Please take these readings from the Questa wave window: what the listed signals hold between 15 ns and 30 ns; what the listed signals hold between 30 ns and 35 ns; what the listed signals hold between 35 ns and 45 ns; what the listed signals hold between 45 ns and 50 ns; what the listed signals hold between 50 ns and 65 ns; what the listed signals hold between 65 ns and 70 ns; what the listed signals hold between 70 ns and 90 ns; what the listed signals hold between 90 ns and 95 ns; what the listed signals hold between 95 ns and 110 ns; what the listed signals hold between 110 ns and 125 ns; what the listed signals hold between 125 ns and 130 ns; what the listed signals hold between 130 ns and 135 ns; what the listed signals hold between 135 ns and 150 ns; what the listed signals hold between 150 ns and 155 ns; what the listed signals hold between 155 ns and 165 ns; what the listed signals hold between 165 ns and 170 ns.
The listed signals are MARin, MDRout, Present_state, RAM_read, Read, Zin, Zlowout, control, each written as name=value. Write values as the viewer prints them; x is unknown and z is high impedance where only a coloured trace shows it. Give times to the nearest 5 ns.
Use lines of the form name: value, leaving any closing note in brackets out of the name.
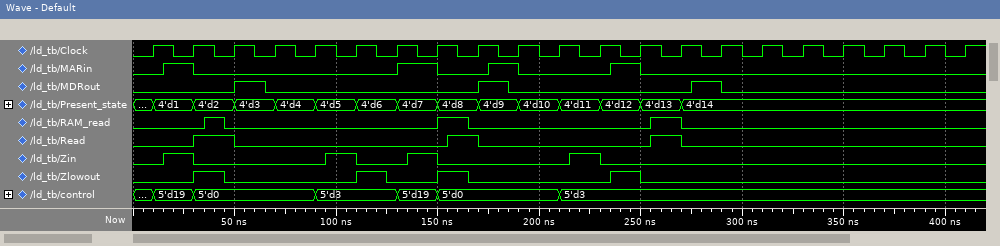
what the listed signals hold between 15 ns and 30 ns: MARin=1, MDRout=0, Present_state=4'd1, RAM_read=0, Read=0, Zin=1, Zlowout=0, control=5'd19
what the listed signals hold between 30 ns and 35 ns: MARin=0, MDRout=0, Present_state=4'd2, RAM_read=0, Read=1, Zin=0, Zlowout=1, control=5'd0
what the listed signals hold between 35 ns and 45 ns: MARin=0, MDRout=0, Present_state=4'd2, RAM_read=1, Read=1, Zin=0, Zlowout=1, control=5'd0
what the listed signals hold between 45 ns and 50 ns: MARin=0, MDRout=0, Present_state=4'd2, RAM_read=0, Read=1, Zin=0, Zlowout=0, control=5'd0
what the listed signals hold between 50 ns and 65 ns: MARin=0, MDRout=1, Present_state=4'd3, RAM_read=0, Read=0, Zin=0, Zlowout=0, control=5'd0
what the listed signals hold between 65 ns and 70 ns: MARin=0, MDRout=0, Present_state=4'd3, RAM_read=0, Read=0, Zin=0, Zlowout=0, control=5'd0
what the listed signals hold between 70 ns and 90 ns: MARin=0, MDRout=0, Present_state=4'd4, RAM_read=0, Read=0, Zin=0, Zlowout=0, control=5'd0
what the listed signals hold between 90 ns and 95 ns: MARin=0, MDRout=0, Present_state=4'd5, RAM_read=0, Read=0, Zin=0, Zlowout=0, control=5'd3
what the listed signals hold between 95 ns and 110 ns: MARin=0, MDRout=0, Present_state=4'd5, RAM_read=0, Read=0, Zin=1, Zlowout=0, control=5'd3
what the listed signals hold between 110 ns and 125 ns: MARin=0, MDRout=0, Present_state=4'd6, RAM_read=0, Read=0, Zin=0, Zlowout=1, control=5'd3
what the listed signals hold between 125 ns and 130 ns: MARin=0, MDRout=0, Present_state=4'd6, RAM_read=0, Read=0, Zin=0, Zlowout=0, control=5'd3
what the listed signals hold between 130 ns and 135 ns: MARin=1, MDRout=0, Present_state=4'd7, RAM_read=0, Read=0, Zin=0, Zlowout=0, control=5'd19
what the listed signals hold between 135 ns and 150 ns: MARin=1, MDRout=0, Present_state=4'd7, RAM_read=0, Read=0, Zin=1, Zlowout=0, control=5'd19
what the listed signals hold between 150 ns and 155 ns: MARin=0, MDRout=0, Present_state=4'd8, RAM_read=1, Read=0, Zin=0, Zlowout=1, control=5'd0
what the listed signals hold between 155 ns and 165 ns: MARin=0, MDRout=0, Present_state=4'd8, RAM_read=1, Read=1, Zin=0, Zlowout=1, control=5'd0
what the listed signals hold between 165 ns and 170 ns: MARin=0, MDRout=0, Present_state=4'd8, RAM_read=0, Read=1, Zin=0, Zlowout=0, control=5'd0
